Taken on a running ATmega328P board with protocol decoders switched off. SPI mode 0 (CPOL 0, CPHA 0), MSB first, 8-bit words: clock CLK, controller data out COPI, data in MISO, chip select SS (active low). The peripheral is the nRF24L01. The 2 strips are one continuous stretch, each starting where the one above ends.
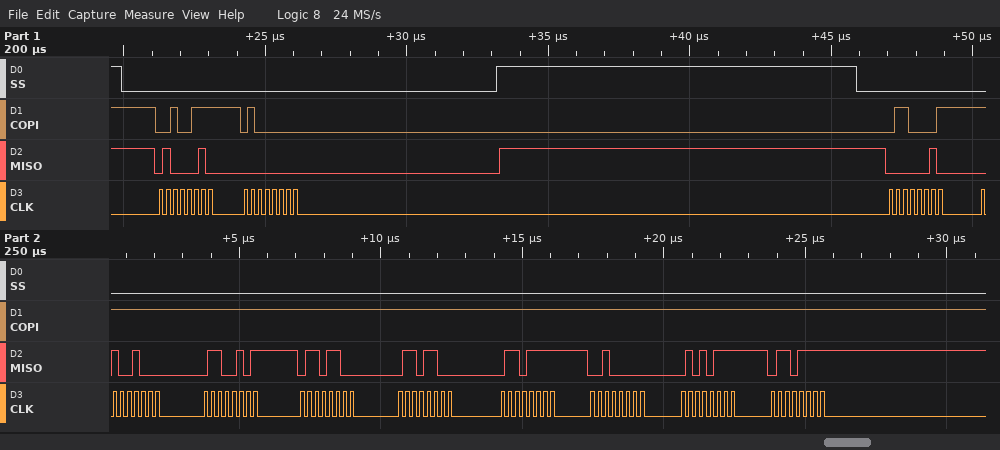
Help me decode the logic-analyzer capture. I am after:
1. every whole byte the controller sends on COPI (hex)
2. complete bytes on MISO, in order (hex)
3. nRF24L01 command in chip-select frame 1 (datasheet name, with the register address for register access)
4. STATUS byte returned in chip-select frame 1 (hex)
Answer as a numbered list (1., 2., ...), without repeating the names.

1. 27 40 61 FF FF FF FF FF FF FF FF
2. 42 00 02 48 65 6C 6C 6F 20 57 6F
3. W_REGISTER 0x07
4. 0x42
